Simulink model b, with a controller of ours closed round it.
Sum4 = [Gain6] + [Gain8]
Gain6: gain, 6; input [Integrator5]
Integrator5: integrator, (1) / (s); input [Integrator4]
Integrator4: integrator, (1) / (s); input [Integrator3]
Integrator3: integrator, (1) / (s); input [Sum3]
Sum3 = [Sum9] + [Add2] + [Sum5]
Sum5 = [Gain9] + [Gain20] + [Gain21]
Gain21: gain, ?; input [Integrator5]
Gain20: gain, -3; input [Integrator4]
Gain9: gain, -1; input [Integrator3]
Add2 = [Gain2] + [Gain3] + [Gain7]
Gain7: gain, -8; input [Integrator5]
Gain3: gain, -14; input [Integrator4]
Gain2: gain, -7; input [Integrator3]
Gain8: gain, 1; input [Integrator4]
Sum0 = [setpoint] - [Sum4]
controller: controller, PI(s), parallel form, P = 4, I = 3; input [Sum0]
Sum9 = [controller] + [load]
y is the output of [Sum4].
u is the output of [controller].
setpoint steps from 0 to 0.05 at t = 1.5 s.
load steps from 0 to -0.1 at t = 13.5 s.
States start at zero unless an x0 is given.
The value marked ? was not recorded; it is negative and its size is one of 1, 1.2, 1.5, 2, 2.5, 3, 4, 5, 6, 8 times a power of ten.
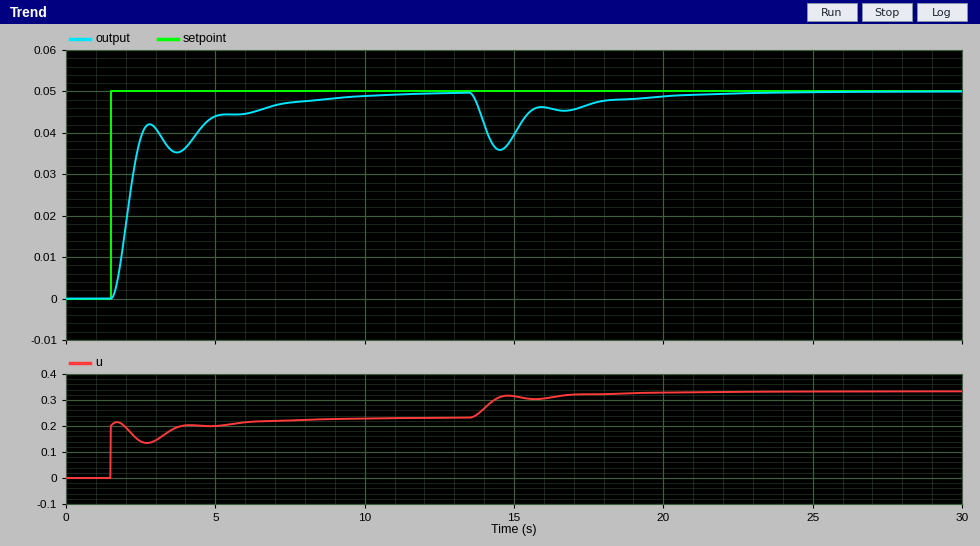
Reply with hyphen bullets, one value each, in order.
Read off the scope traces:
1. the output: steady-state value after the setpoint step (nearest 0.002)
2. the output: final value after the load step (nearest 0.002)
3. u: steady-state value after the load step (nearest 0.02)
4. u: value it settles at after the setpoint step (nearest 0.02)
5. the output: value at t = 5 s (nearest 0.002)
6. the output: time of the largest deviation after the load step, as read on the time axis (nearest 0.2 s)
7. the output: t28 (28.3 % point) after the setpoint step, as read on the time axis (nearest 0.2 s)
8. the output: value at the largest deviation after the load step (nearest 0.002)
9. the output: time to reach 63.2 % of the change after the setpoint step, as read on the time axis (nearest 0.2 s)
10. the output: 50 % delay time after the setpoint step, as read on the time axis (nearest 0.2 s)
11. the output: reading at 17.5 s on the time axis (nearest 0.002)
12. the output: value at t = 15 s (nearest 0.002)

- 0.050
- 0.050
- 0.34
- 0.24
- 0.044
- 14.6 s
- 2.0 s
- 0.036
- 2.2 s
- 2.2 s
- 0.046
- 0.040
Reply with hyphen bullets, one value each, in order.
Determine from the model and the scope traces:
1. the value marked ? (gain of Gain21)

- -20
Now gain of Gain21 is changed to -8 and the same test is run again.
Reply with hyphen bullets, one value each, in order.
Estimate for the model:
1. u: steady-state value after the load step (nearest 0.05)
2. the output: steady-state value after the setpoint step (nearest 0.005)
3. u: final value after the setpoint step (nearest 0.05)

- 0.25
- 0.050
- 0.15
